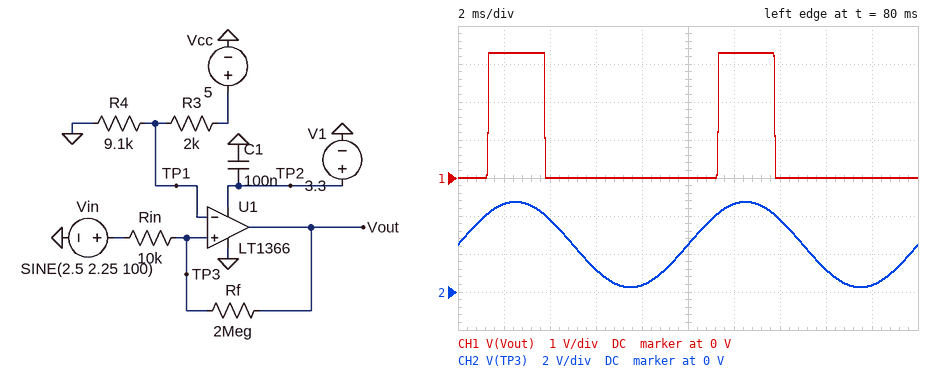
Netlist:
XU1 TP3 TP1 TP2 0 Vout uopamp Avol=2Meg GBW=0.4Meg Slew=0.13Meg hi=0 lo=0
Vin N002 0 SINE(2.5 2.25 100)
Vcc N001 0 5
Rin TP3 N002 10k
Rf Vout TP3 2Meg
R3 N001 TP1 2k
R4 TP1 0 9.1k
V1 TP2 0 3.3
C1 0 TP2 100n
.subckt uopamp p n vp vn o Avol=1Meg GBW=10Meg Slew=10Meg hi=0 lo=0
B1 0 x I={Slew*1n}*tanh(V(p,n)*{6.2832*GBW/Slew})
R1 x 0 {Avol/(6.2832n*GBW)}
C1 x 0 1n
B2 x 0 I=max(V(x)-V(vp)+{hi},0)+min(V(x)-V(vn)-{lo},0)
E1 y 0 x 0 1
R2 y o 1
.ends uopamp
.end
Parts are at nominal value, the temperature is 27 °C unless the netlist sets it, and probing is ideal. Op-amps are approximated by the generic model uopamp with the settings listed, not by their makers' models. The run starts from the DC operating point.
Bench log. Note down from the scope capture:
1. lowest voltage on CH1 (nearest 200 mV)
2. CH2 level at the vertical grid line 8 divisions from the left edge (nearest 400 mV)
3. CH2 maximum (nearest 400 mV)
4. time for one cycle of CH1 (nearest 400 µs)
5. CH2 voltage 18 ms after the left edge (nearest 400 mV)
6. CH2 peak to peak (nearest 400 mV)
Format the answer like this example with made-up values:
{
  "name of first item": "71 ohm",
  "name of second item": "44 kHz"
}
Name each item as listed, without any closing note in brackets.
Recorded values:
{
  "lowest voltage on CH1": "0 V",
  "CH2 level at the vertical grid line 8 divisions from the left edge": "1.2 V",
  "CH2 maximum": "4.8 V",
  "time for one cycle of CH1": "10.0 ms",
  "CH2 voltage 18 ms after the left edge": "400 mV",
  "CH2 peak to peak": "4.4 V"
}
